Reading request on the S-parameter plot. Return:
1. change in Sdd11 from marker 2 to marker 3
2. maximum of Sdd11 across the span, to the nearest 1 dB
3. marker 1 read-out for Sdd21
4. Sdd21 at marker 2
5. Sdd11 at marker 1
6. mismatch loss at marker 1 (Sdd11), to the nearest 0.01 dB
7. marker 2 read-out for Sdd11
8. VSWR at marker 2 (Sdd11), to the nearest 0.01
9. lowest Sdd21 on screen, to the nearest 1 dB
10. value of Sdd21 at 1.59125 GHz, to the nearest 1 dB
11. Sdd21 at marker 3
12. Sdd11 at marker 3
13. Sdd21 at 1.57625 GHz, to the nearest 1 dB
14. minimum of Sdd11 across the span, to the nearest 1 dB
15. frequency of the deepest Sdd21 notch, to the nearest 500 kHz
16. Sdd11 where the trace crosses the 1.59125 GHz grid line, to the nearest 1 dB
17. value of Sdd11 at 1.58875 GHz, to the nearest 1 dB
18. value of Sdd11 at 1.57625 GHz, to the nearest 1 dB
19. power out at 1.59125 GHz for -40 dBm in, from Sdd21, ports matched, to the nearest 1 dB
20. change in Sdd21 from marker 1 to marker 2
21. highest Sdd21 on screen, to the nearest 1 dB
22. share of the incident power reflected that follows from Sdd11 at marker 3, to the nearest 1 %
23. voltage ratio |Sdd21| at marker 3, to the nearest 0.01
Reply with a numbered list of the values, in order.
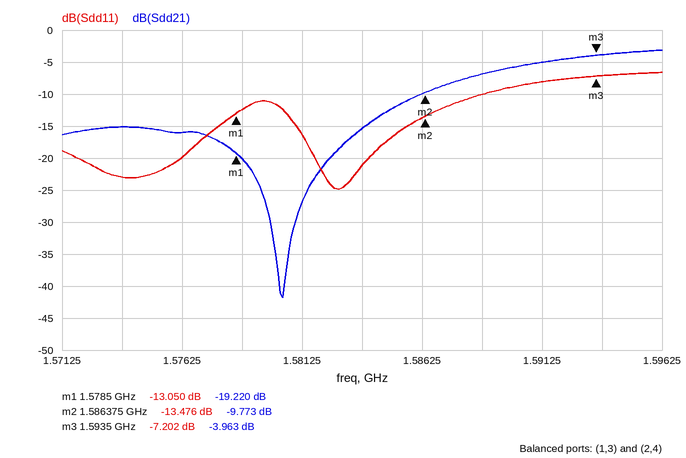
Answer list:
1. 6.274 dB
2. -7 dB
3. -19.220 dB
4. -9.773 dB
5. -13.050 dB
6. 0.22 dB
7. -13.476 dB
8. 1.54
9. -42 dB
10. -5 dB
11. -3.963 dB
12. -7.202 dB
13. -16 dB
14. -25 dB
15. 1.5805 GHz
16. -8 dB
17. -10 dB
18. -20 dB
19. -45 dBm
20. 9.447 dB
21. -3 dB
22. 19 %
23. 0.63
